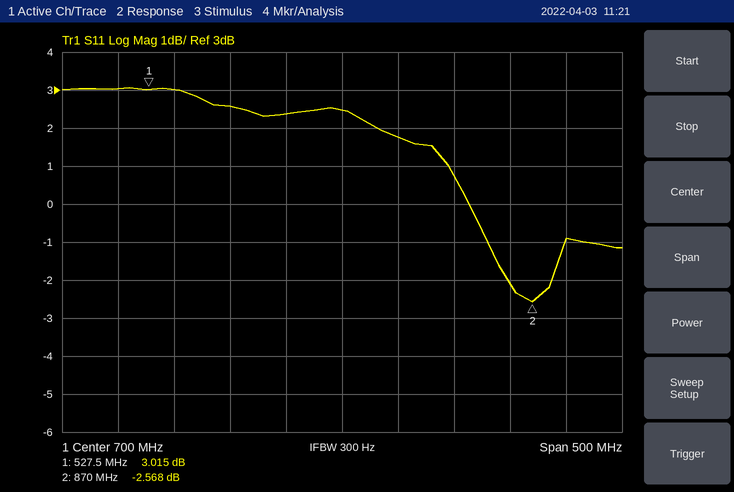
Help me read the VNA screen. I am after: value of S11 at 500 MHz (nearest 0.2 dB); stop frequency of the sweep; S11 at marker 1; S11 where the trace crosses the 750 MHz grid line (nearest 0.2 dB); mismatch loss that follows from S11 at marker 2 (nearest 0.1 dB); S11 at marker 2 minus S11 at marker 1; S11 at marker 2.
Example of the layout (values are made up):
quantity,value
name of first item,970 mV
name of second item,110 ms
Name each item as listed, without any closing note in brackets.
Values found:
quantity,value
value of S11 at 500 MHz,3.0 dB
stop frequency of the sweep,950 MHz
S11 at marker 1,3.015 dB
S11 where the trace crosses the 750 MHz grid line,1.8 dB
mismatch loss that follows from S11 at marker 2,3.5 dB
S11 at marker 2 minus S11 at marker 1,-5.583 dB
S11 at marker 2,-2.568 dB
